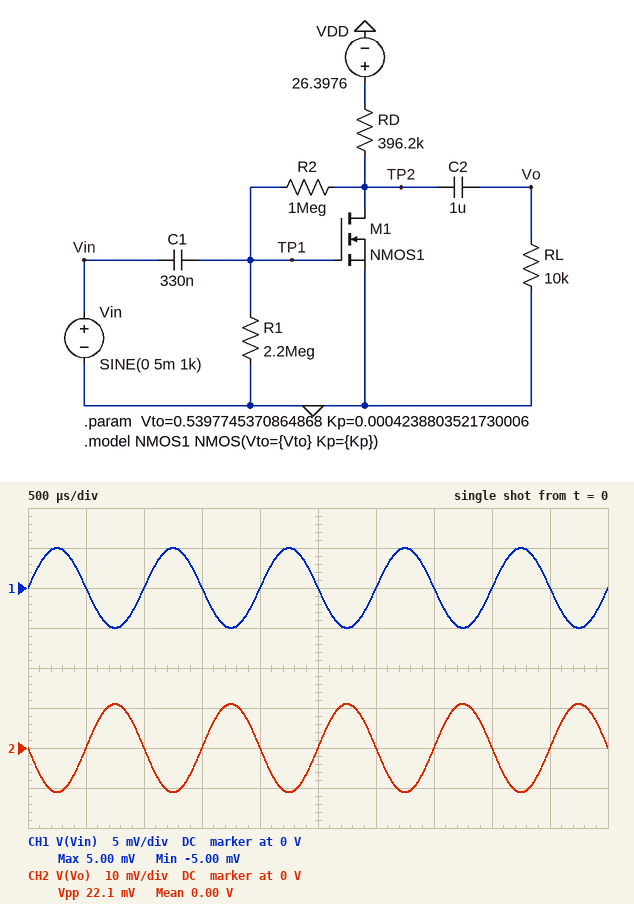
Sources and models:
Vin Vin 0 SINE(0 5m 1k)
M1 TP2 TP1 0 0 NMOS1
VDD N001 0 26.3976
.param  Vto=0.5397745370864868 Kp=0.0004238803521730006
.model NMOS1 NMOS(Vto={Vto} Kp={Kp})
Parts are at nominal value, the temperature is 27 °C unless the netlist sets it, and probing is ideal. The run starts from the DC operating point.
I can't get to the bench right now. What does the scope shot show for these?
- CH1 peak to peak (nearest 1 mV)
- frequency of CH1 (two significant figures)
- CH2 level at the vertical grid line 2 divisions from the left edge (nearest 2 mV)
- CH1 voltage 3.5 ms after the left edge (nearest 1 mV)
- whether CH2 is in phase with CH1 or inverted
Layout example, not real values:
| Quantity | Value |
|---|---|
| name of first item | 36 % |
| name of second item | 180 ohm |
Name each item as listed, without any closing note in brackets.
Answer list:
| Quantity | Value |
|---|---|
| CH1 peak to peak | 10 mV |
| frequency of CH1 | 1.0 kHz |
| CH2 level at the vertical grid line 2 divisions from the left edge | 0 V |
| CH1 voltage 3.5 ms after the left edge | 0 V |
| whether CH2 is in phase with CH1 or inverted | inverted |
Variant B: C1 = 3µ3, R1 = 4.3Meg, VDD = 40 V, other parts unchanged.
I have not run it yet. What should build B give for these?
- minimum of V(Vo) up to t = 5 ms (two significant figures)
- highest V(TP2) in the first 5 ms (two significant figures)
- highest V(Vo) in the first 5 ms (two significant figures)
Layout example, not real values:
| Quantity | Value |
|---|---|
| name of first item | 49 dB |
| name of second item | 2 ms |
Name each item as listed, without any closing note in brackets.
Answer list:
| Quantity | Value |
|---|---|
| minimum of V(Vo) up to t = 5 ms | -14 mV |
| highest V(TP2) in the first 5 ms | 1.5 V |
| highest V(Vo) in the first 5 ms | 14 mV |
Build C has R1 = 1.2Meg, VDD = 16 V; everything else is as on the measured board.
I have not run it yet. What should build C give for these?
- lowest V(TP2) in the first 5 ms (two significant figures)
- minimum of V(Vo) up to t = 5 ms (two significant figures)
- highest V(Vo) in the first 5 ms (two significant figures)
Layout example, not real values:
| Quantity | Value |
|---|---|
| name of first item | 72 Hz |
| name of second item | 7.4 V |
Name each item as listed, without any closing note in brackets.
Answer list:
| Quantity | Value |
|---|---|
| lowest V(TP2) in the first 5 ms | 1.7 V |
| minimum of V(Vo) up to t = 5 ms | -8.3 mV |
| highest V(Vo) in the first 5 ms | 8.3 mV |
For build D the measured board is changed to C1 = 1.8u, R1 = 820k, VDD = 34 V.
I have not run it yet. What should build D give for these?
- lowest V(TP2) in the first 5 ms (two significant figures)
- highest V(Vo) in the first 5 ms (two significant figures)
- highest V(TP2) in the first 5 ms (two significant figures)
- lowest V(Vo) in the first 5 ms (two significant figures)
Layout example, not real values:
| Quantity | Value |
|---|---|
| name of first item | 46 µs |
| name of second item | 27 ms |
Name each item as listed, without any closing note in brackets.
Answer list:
| Quantity | Value |
|---|---|
| lowest V(TP2) in the first 5 ms | 2.5 V |
| highest V(Vo) in the first 5 ms | 12 mV |
| highest V(TP2) in the first 5 ms | 2.6 V |
| lowest V(Vo) in the first 5 ms | -12 mV |
